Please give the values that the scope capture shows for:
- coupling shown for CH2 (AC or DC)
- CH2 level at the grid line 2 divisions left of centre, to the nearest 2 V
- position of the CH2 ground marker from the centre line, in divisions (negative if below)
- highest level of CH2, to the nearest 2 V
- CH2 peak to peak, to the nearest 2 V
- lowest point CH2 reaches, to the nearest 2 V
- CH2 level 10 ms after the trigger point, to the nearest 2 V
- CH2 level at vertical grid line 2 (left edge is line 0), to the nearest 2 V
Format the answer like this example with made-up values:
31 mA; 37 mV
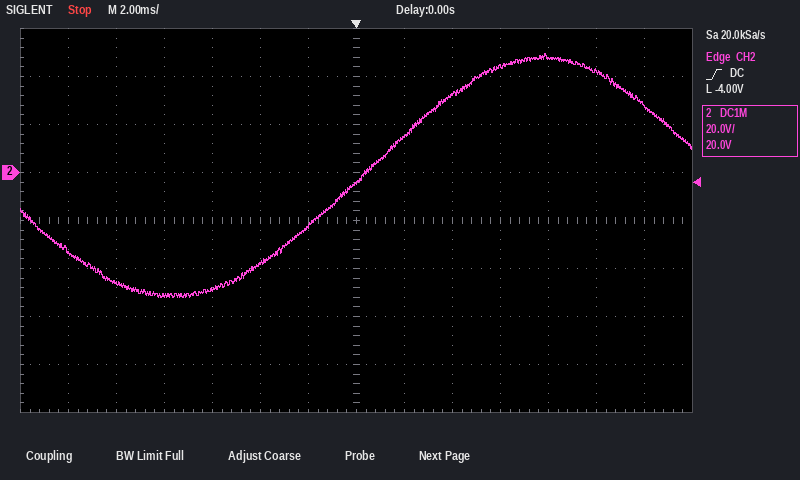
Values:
DC; -38 V; +1.0 div; 50 V; 102 V; -52 V; 42 V; -46 V
